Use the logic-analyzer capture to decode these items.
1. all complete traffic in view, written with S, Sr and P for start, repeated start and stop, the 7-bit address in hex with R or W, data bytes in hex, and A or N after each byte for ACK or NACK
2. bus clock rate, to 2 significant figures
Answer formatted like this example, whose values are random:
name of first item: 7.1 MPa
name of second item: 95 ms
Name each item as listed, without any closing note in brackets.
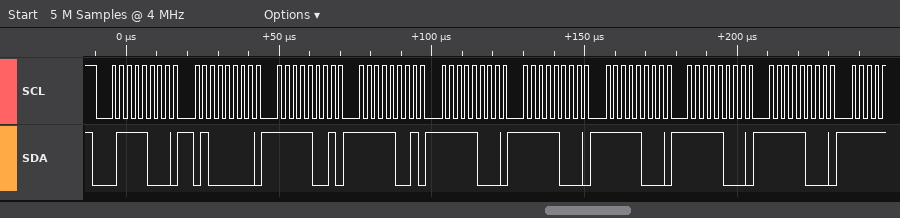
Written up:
all complete traffic in view, written with S, Sr and P for start, repeated start and stop, the 7-bit address in hex with R or W, data bytes in hex, and A or N after each byte for ACK or NACK: S 3CW A 40 A F9 A F9 A F8 A F8 A F8 A F8 A F8 A
bus clock rate, to 2 significant figures: 400 kHz
